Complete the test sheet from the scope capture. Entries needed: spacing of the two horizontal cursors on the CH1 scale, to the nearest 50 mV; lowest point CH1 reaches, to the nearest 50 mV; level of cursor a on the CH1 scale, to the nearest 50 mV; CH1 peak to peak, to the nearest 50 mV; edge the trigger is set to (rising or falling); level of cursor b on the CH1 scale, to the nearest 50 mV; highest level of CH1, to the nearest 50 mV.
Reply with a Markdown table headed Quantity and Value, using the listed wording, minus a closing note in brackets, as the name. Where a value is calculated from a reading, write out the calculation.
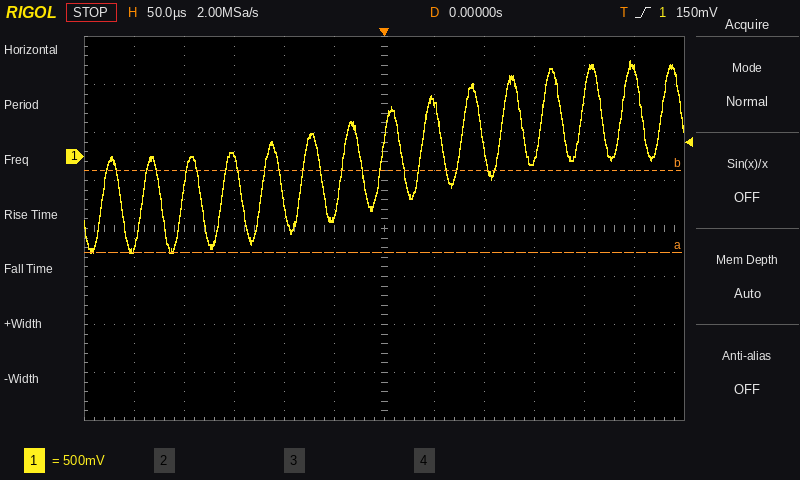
| Quantity | Value |
|---|---|
| spacing of the two horizontal cursors on the CH1 scale, to the nearest 50 mV | 850 mV |
| lowest point CH1 reaches, to the nearest 50 mV | -1.00 V |
| level of cursor a on the CH1 scale, to the nearest 50 mV | -1.00 V |
| CH1 peak to peak, to the nearest 50 mV | 1.00 V − (-1.00 V) = 2.00 V |
| edge the trigger is set to | rising |
| level of cursor b on the CH1 scale, to the nearest 50 mV | -150 mV |
| highest level of CH1, to the nearest 50 mV | 1.00 V |
